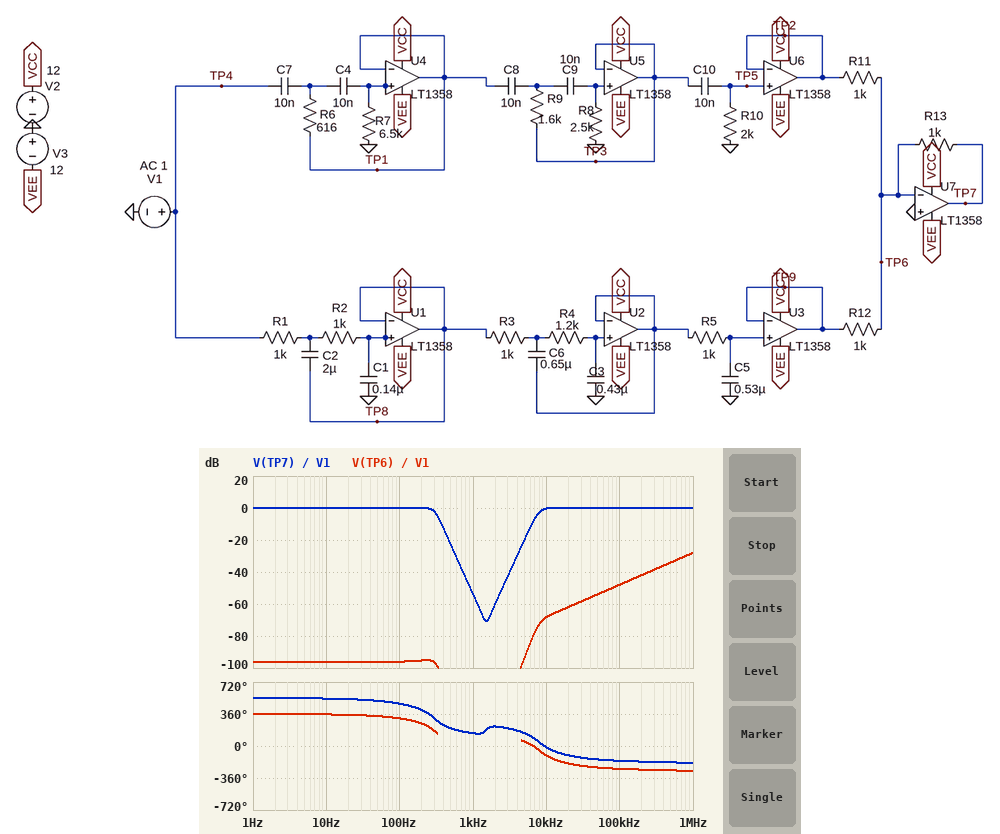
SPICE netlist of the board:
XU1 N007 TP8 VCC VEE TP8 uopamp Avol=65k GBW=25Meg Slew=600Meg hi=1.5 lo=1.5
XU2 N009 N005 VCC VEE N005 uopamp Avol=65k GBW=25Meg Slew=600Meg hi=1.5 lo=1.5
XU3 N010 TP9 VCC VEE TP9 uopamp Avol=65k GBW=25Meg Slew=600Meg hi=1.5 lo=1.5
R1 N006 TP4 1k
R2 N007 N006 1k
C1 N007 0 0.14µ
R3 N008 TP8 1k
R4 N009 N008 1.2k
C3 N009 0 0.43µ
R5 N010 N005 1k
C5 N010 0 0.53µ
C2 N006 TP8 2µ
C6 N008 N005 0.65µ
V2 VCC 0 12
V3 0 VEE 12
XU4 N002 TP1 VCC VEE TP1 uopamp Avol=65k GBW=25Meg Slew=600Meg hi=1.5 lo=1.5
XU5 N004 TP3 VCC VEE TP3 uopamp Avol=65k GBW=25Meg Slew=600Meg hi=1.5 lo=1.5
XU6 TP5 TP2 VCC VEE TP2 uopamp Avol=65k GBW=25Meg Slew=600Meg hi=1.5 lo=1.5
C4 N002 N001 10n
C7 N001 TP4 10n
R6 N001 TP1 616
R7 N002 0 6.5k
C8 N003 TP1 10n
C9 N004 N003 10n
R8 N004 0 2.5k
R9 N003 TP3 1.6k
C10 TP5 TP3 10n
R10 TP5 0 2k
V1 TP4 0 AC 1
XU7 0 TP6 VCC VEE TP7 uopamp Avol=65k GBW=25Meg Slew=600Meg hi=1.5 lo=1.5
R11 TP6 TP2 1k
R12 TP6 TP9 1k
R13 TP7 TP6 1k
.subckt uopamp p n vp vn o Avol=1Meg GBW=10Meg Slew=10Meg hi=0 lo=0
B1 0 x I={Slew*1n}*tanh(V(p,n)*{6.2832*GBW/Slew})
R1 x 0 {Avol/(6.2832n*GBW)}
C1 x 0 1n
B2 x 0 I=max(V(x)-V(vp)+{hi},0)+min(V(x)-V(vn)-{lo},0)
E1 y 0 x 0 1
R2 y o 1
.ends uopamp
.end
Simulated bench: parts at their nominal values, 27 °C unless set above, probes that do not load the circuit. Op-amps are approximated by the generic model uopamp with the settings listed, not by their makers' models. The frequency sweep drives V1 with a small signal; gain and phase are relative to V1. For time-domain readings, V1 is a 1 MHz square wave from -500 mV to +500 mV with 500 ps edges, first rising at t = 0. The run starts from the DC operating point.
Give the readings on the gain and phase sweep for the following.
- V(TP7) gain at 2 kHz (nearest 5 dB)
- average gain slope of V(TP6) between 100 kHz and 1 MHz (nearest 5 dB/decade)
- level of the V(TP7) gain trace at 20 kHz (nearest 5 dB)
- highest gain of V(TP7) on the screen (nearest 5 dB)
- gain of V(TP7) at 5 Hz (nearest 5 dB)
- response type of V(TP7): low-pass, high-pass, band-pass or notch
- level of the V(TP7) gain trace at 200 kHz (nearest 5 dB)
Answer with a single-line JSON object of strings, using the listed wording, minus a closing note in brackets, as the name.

{"V(TP7) gain at 2 kHz": "-60 dB", "average gain slope of V(TP6) between 100 kHz and 1 MHz": "20 dB/decade", "level of the V(TP7) gain trace at 20 kHz": "0 dB", "highest gain of V(TP7) on the screen": "0 dB", "gain of V(TP7) at 5 Hz": "0 dB", "response type of V(TP7): low-pass, high-pass, band-pass or notch": "notch", "level of the V(TP7) gain trace at 200 kHz": "0 dB"}
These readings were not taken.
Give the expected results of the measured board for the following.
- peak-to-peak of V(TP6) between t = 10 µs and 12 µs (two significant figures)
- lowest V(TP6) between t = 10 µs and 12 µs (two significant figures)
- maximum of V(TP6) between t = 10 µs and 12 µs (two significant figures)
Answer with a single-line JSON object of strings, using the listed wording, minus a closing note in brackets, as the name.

{"peak-to-peak of V(TP6) between t = 10 µs and 12 µs": "300 mV", "lowest V(TP6) between t = 10 µs and 12 µs": "-150 mV", "maximum of V(TP6) between t = 10 µs and 12 µs": "150 mV"}
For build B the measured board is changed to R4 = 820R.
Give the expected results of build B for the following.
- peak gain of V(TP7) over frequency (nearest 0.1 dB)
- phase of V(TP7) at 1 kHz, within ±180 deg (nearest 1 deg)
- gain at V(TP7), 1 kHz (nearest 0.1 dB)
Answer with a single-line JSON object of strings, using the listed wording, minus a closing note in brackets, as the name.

{"peak gain of V(TP7) over frequency": "0.8 dB", "phase of V(TP7) at 1 kHz, within ±180 deg": "149 deg", "gain at V(TP7), 1 kHz": "-50.5 dB"}
